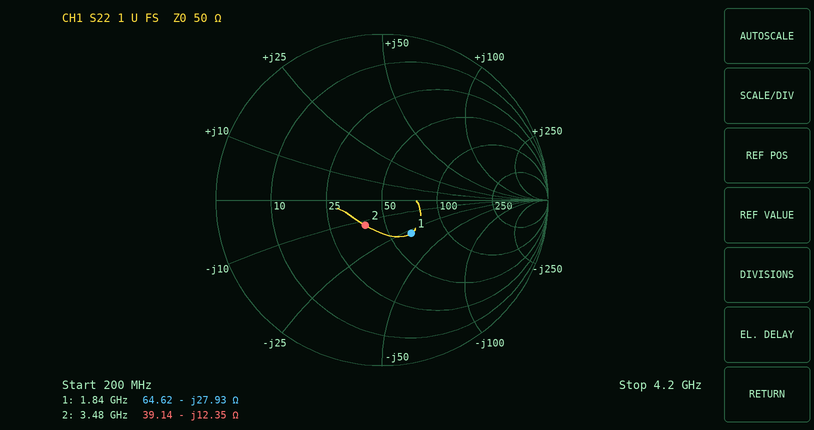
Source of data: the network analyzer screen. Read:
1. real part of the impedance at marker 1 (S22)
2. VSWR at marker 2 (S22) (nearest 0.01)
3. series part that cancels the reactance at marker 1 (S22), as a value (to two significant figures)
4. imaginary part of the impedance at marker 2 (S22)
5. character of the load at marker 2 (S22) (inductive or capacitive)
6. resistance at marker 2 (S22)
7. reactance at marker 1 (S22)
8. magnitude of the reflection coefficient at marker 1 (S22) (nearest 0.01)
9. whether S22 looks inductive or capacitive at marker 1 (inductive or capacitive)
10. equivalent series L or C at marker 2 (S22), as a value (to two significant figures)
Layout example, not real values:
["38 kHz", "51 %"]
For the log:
["64.62 Ω", "1.45", "2.4 nH", "-12.35 Ω", "capacitive", "39.14 Ω", "-27.93 Ω", "0.27", "capacitive", "3.7 pF"]
